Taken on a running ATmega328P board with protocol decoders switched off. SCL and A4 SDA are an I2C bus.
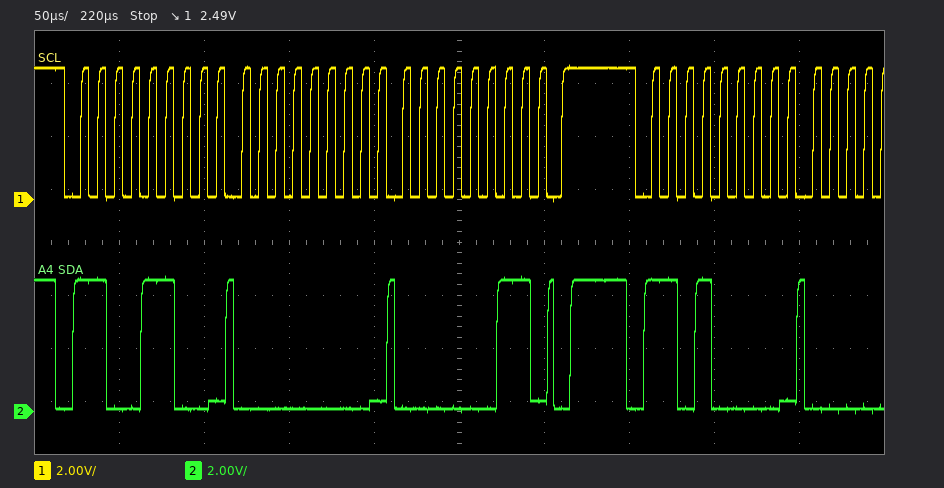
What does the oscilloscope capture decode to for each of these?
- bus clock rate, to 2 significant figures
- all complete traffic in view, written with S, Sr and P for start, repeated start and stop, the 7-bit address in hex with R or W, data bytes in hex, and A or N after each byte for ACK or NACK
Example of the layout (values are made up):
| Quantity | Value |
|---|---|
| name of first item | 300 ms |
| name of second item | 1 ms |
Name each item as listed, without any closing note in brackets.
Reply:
| Quantity | Value |
|---|---|
| bus clock rate, to 2 significant figures | 100 kHz |
| all complete traffic in view, written with S, Sr and P for start, repeated start and stop, the 7-bit address in hex with R or W, data bytes in hex, and A or N after each byte for ACK or NACK | S 66W A 00 A 03 A P S 68W A |
